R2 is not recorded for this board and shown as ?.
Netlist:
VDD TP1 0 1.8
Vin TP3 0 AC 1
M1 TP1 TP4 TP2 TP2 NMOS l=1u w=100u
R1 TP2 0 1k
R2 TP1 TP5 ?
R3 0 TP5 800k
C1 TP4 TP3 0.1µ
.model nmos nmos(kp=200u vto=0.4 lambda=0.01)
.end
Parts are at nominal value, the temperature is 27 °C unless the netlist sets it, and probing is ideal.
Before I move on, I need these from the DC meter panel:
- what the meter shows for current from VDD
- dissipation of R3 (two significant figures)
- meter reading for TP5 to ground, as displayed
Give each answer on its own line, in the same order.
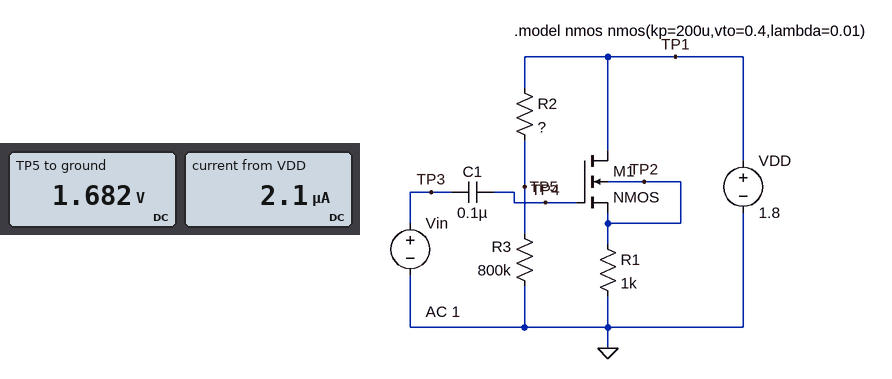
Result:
2.1 µA
3.5 µW
1.682 V
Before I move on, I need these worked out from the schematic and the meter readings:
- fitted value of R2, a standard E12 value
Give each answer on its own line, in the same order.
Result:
56 kΩ
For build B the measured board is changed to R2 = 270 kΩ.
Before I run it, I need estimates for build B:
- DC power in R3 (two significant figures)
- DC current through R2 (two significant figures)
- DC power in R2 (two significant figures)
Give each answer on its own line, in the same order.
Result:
2.3 µW
1.7 µA
760 nW
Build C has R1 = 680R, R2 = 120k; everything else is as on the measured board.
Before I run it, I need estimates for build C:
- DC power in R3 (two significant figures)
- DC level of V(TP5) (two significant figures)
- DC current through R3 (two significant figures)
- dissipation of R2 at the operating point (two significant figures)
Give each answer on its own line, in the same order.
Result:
3.1 µW
1.6 V
2.0 µA
460 nW
